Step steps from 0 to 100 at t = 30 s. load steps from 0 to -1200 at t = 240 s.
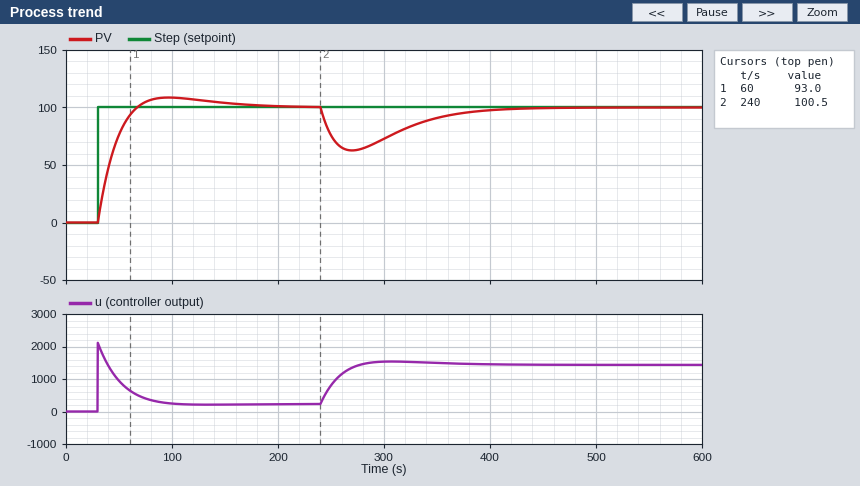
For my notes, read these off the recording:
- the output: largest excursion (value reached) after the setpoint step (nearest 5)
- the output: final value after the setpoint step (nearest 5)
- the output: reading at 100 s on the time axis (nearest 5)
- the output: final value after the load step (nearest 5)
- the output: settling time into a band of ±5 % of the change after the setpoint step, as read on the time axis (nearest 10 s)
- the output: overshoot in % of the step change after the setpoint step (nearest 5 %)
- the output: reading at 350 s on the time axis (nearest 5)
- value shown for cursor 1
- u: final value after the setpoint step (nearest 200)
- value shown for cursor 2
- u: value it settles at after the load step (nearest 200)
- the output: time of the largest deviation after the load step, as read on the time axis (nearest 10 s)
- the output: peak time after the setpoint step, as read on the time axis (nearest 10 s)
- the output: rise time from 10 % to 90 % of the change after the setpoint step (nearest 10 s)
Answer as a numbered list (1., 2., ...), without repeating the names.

1. 110
2. 100
3. 110
4. 100
5. 140 s
6. 10 %
7. 90
8. 93.0
9. 200
10. 100.5
11. 1400
12. 270 s
13. 100 s
14. 30 s
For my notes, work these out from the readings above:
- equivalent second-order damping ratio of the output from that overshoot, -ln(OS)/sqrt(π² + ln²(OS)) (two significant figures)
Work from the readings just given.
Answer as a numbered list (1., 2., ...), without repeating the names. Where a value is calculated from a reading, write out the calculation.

1. ln(0.1) = -2.303; 2.303 / sqrt(9.870 + 5.302) = 0.59
